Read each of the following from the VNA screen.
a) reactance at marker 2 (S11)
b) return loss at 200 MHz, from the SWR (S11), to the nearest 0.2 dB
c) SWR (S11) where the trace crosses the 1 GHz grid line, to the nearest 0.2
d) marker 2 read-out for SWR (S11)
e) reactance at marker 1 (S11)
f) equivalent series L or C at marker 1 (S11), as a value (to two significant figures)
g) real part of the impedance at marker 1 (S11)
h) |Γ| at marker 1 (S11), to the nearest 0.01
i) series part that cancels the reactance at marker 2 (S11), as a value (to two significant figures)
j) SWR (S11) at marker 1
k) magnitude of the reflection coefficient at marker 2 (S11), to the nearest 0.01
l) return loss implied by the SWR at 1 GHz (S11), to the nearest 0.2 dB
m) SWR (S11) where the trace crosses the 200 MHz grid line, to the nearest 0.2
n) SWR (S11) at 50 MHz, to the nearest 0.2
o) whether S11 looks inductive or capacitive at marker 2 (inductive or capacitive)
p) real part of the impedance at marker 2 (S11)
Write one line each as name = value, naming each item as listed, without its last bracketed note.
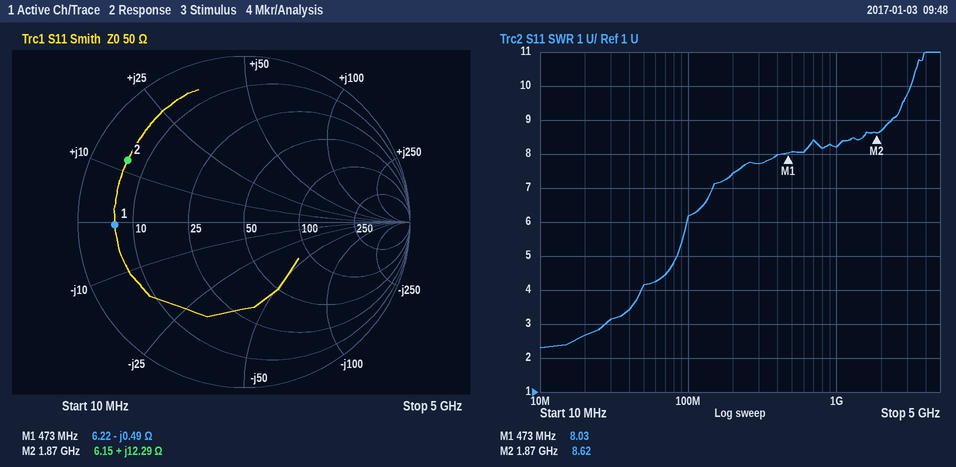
reactance at marker 2 = +12.29 Ω
return loss at 200 MHz, from the SWR (S11), to the nearest 0.2 dB = 2.4 dB
SWR (S11) where the trace crosses the 1 GHz grid line, to the nearest 0.2 = 8.2
marker 2 read-out for SWR = 8.62
reactance at marker 1 = -0.49 Ω
equivalent series L or C at marker 1 (S11), as a value = 690 pF
real part of the impedance at marker 1 = 6.22 Ω
|Γ| at marker 1 (S11), to the nearest 0.01 = 0.78
series part that cancels the reactance at marker 2 (S11), as a value = 6.9 pF
SWR (S11) at marker 1 = 8.03
magnitude of the reflection coefficient at marker 2 (S11), to the nearest 0.01 = 0.79
return loss implied by the SWR at 1 GHz (S11), to the nearest 0.2 dB = 2.2 dB
SWR (S11) where the trace crosses the 200 MHz grid line, to the nearest 0.2 = 7.4
SWR (S11) at 50 MHz, to the nearest 0.2 = 4.2
whether S11 looks inductive or capacitive at marker 2 = inductive
real part of the impedance at marker 2 = 6.15 Ω
